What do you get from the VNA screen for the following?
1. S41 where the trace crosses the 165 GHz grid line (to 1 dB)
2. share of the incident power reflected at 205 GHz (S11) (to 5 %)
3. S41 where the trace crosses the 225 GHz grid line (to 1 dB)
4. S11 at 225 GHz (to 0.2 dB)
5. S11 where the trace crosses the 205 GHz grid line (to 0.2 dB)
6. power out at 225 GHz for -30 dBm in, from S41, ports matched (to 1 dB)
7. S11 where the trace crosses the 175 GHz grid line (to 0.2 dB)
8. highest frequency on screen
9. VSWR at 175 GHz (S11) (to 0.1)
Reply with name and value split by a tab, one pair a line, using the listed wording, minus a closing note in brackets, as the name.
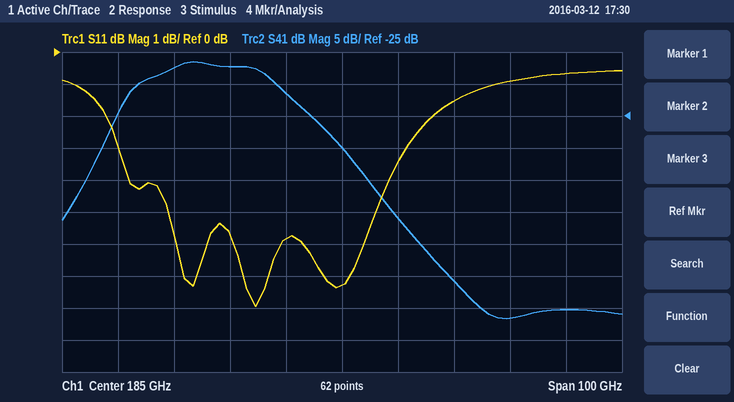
S41 where the trace crosses the 165 GHz grid line	-17 dB
share of the incident power reflected at 205 GHz (S11)	70 %
S41 where the trace crosses the 225 GHz grid line	-55 dB
S11 at 225 GHz	-0.6 dB
S11 where the trace crosses the 205 GHz grid line	-1.6 dB
power out at 225 GHz for -30 dBm in, from S41, ports matched	-85 dBm
S11 where the trace crosses the 175 GHz grid line	-5.8 dB
highest frequency on screen	235 GHz
VSWR at 175 GHz (S11)	3.1
